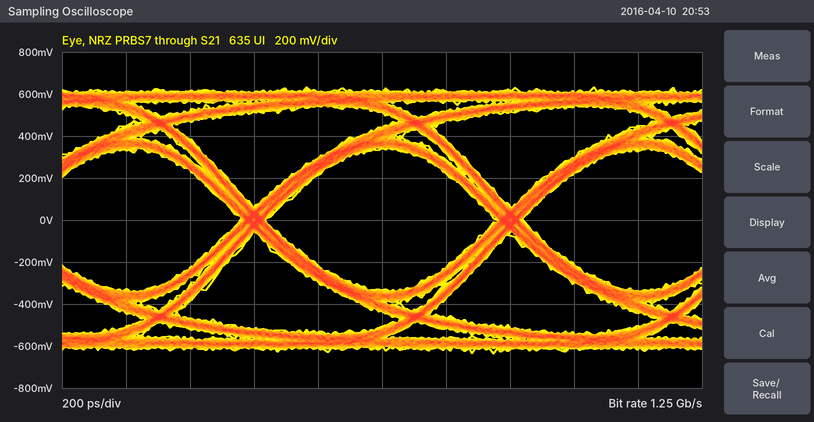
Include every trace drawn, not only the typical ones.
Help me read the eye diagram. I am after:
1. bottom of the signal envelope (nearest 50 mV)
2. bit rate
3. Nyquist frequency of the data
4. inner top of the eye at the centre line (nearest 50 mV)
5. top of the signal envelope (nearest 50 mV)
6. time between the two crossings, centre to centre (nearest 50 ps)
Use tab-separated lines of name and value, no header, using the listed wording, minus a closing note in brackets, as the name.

bottom of the signal envelope	-650 mV
bit rate	1.25 Gb/s
Nyquist frequency of the data	625 MHz
inner top of the eye at the centre line	350 mV
top of the signal envelope	650 mV
time between the two crossings, centre to centre	800 ps
